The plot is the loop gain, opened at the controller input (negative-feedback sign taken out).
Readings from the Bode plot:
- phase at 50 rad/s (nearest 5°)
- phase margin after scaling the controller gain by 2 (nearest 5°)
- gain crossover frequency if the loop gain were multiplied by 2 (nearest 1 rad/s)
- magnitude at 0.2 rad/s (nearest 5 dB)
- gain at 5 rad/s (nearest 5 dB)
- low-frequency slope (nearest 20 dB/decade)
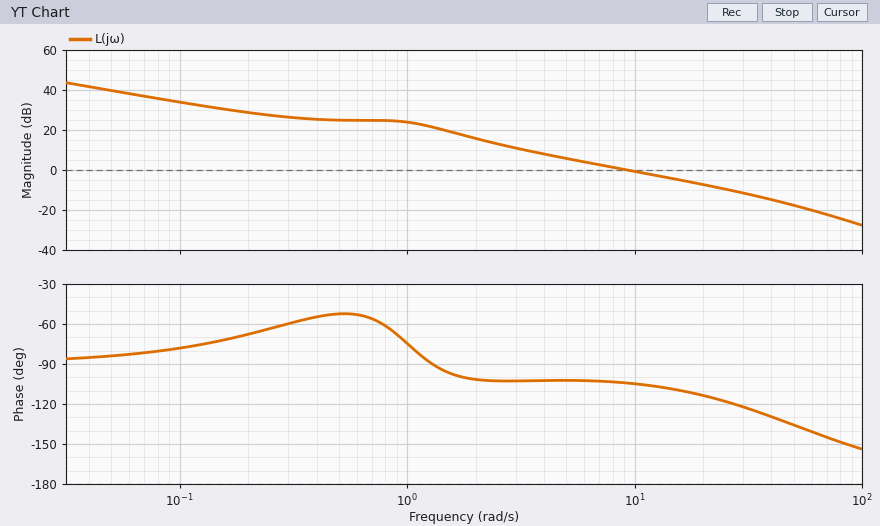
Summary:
-135°
70°
18 rad/s
30 dB
5 dB
-20 dB/decade
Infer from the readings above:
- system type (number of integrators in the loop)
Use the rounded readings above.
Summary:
1
